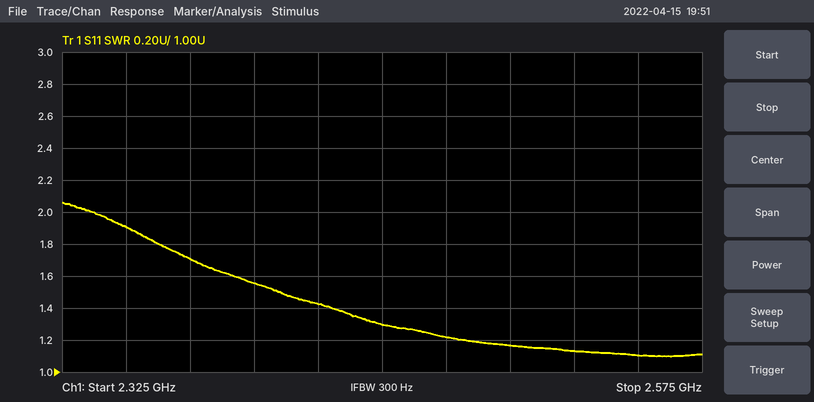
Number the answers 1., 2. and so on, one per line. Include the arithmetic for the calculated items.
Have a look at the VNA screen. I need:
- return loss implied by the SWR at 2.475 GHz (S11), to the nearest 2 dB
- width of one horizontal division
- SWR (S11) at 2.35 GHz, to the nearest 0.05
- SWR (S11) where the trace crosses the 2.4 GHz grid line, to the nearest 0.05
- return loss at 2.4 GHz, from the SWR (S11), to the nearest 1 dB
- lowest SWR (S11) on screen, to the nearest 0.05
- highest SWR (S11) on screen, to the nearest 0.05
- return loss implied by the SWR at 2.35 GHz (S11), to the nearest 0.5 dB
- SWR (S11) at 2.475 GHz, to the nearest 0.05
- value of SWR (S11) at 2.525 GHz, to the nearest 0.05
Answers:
1. −20 log10((1.2 − 1)/(1.2 + 1)) ≈ 20.8 dB, so 20 dB to the nearest 2 dB
2. 25 MHz
3. 1.90
4. 1.55
5. −20 log10((1.55 − 1)/(1.55 + 1)) ≈ 13 dB
6. 1.10
7. 2.05
8. −20 log10((1.9 − 1)/(1.9 + 1)) ≈ 10.2 dB, so 10.0 dB to the nearest 0.5 dB
9. 1.20
10. 1.15
